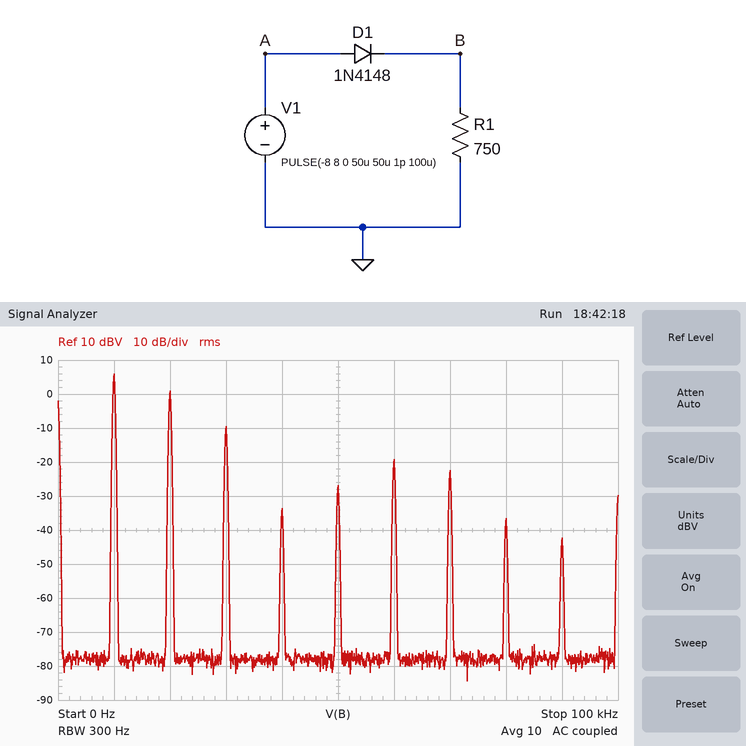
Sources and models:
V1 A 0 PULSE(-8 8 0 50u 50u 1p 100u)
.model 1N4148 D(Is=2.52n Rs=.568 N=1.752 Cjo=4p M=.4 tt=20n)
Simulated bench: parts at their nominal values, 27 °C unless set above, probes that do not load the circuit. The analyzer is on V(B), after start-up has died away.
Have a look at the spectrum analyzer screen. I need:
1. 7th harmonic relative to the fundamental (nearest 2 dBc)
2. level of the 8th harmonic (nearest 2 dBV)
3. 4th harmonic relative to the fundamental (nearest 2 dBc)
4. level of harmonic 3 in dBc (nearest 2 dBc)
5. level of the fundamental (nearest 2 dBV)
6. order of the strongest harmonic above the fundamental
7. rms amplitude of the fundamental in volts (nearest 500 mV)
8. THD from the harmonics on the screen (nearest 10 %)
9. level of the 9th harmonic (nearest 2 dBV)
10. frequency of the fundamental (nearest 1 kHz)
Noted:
-28 dBc
-36 dBV
-40 dBc
-16 dBc
6 dBV
2
2.0 V
60 %
-42 dBV
10 kHz
